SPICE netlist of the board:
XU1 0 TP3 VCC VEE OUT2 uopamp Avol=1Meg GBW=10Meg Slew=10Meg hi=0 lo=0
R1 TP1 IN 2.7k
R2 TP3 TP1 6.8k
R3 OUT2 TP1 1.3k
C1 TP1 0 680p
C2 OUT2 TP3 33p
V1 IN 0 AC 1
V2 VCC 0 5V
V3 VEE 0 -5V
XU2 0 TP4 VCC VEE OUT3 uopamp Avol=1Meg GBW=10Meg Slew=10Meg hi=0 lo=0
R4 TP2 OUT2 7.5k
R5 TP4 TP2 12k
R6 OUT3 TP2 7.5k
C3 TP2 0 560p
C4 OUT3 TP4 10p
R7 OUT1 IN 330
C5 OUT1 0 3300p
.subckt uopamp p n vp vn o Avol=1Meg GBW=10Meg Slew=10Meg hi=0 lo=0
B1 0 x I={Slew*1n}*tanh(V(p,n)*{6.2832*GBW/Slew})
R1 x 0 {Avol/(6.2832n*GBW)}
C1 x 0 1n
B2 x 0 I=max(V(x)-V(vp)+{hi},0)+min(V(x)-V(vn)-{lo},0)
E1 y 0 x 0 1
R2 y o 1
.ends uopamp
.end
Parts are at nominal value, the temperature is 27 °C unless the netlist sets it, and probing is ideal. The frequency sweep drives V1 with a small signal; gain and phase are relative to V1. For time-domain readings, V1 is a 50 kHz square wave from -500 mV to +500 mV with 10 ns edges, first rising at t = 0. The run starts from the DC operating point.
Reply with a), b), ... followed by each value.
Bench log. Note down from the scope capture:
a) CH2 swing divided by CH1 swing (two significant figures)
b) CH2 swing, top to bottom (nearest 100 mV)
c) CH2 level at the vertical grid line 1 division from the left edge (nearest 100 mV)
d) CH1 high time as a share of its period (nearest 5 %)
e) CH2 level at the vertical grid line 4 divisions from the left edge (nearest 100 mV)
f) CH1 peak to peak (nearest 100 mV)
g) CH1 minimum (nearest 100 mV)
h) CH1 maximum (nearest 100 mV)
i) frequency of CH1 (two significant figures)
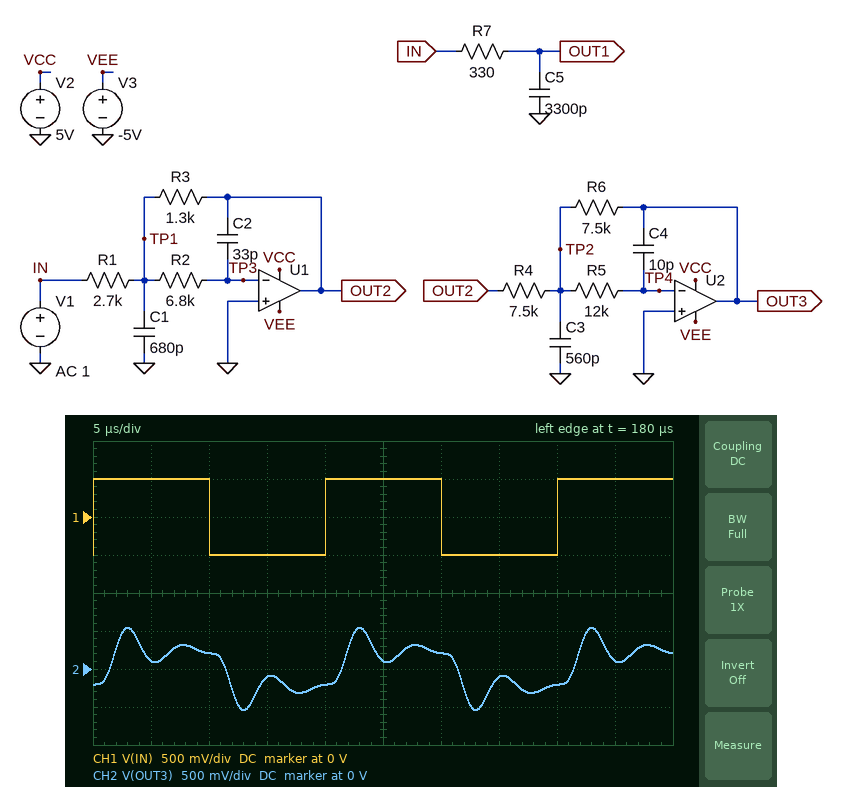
a) 1.1
b) 1.1 V
c) 100 mV
d) 50 %
e) -200 mV
f) 1.0 V
g) -500 mV
h) 500 mV
i) 50 kHz
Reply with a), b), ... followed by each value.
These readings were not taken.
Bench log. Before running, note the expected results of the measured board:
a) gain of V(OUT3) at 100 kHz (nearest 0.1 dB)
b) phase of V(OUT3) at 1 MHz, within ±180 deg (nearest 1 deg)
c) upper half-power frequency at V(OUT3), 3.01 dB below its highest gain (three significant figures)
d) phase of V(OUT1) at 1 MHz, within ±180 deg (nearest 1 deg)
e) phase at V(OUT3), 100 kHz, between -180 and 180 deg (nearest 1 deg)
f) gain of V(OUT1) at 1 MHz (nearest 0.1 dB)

a) -4.0 dB
b) 13 deg
c) 248 kHz
d) -82 deg
e) -31 deg
f) -16.8 dB
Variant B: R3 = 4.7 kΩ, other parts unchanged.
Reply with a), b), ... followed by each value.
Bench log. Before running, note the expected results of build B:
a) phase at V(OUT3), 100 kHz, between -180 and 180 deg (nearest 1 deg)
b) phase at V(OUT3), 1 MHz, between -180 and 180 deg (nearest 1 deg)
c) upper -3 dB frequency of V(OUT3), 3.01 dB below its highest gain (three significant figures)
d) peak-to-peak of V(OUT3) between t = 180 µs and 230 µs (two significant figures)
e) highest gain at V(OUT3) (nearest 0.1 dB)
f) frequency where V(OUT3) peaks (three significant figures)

a) -52 deg
b) 5 deg
c) 223 kHz
d) 3.7 V
e) 12.4 dB
f) 184 kHz
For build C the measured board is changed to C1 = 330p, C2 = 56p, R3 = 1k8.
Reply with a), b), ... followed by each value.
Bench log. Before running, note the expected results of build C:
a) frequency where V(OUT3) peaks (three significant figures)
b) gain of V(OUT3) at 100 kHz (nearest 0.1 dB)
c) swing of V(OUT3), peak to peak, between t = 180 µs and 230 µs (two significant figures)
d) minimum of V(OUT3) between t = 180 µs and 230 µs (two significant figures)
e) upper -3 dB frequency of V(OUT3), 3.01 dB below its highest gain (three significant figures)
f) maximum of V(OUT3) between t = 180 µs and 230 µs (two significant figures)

a) 196 kHz
b) -1.8 dB
c) 1.2 V
d) -610 mV
e) 237 kHz
f) 610 mV
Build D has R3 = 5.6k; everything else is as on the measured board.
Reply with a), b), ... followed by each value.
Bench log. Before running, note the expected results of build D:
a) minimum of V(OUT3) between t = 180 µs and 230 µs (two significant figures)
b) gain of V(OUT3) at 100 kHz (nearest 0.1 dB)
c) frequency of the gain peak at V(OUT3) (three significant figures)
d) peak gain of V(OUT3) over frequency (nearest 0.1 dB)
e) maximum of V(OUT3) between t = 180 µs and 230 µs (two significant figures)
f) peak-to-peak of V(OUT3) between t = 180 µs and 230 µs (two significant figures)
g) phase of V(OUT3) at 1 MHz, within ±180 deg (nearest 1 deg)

a) -2.1 V
b) 9.6 dB
c) 176 kHz
d) 12.7 dB
e) 2.1 V
f) 4.2 V
g) 4 deg
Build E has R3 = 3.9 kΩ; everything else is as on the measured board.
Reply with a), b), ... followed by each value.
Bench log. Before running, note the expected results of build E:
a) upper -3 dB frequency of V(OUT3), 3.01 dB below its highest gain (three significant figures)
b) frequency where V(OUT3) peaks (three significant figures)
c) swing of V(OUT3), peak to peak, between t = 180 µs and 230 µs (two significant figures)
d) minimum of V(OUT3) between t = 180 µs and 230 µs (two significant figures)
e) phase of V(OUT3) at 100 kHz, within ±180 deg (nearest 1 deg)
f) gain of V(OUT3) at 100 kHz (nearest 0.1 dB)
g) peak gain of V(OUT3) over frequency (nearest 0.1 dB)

a) 227 kHz
b) 190 kHz
c) 3.2 V
d) -1.6 V
e) -47 deg
f) 6.3 dB
g) 11.8 dB
